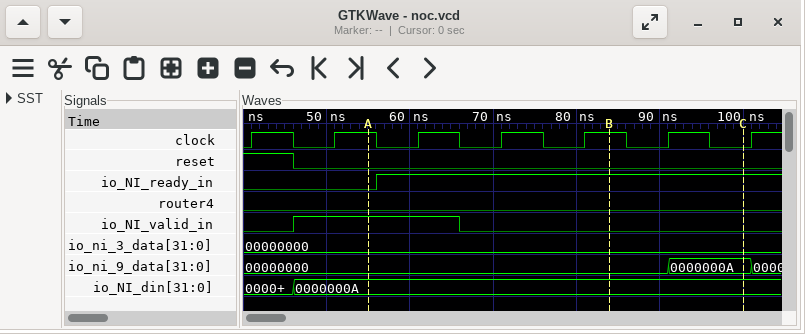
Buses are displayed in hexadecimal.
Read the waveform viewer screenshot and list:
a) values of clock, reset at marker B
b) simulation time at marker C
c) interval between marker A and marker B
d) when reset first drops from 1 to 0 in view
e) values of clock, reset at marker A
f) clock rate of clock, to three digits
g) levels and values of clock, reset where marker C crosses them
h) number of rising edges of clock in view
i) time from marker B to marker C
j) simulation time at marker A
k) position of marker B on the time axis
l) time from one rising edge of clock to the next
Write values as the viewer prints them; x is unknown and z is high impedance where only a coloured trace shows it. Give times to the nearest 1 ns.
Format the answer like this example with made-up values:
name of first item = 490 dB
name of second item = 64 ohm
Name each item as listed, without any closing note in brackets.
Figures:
values of clock, reset at marker B = clock=1, reset=0
simulation time at marker C = 100 ns
interval between marker A and marker B = 29 ns
when reset first drops from 1 to 0 in view = 46 ns
values of clock, reset at marker A = clock=1, reset=0
clock rate of clock, to three digits = 100 MHz
levels and values of clock, reset where marker C crosses them = clock=0, reset=0
number of rising edges of clock in view = 7
time from marker B to marker C = 16 ns
simulation time at marker A = 55 ns
position of marker B on the time axis = 84 ns
time from one rising edge of clock to the next = 10 ns
